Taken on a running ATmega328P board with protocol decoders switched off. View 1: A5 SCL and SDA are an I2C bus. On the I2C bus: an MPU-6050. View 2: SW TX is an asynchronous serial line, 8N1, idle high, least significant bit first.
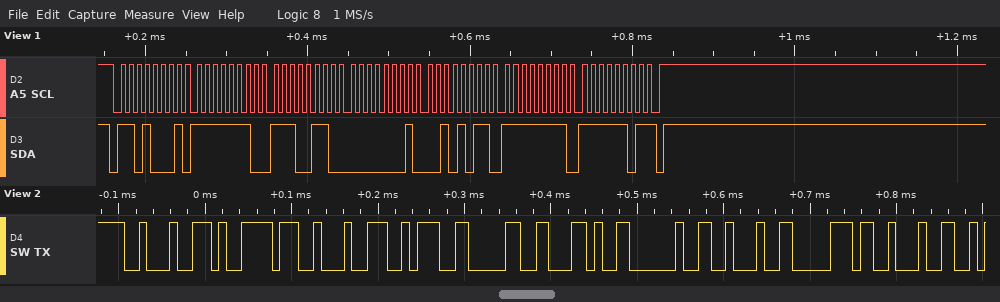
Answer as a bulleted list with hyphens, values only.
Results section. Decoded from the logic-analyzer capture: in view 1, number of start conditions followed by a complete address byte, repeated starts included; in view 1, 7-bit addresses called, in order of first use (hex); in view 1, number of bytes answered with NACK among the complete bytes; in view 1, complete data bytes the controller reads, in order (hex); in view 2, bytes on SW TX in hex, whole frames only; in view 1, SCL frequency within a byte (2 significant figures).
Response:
- 1
- 0x68
- 1
- FE E6 01 2B FF FD
- 22 79 22 3A 30 2C 20 22 70 22
- 100 kHz
